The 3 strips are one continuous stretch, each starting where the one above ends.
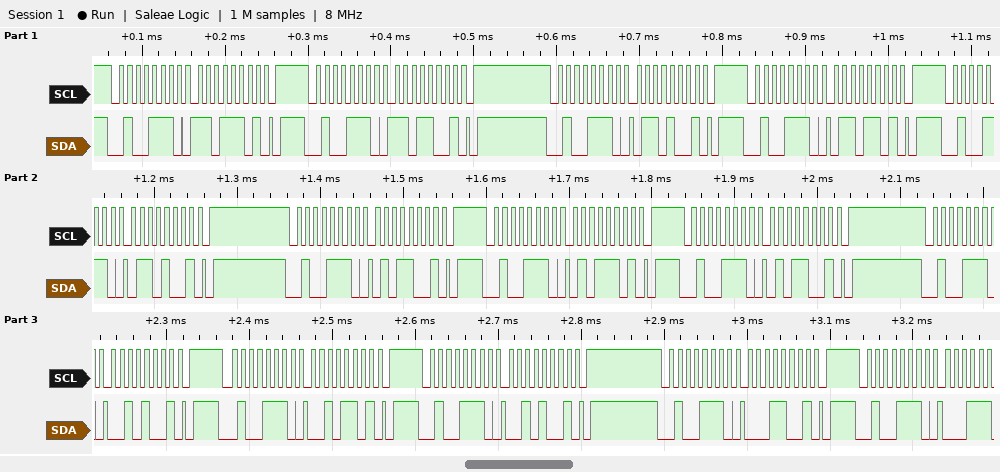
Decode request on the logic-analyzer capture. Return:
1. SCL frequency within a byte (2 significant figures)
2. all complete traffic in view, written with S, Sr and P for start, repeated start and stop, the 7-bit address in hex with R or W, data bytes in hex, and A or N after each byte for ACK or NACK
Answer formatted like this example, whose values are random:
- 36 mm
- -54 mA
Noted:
- 100 kHz
- S 27W A DD A P S 27W A D9 A P S 27W A 69 A P S 27W A 6D A P S 27W A 69 A P S 27W A 59 A P S 27W A 5D A P S 27W A 59 A P S 27W A 29 A P S 27W A 2D A P S 27W A 29 A P S 27W A 19 A P S 27W A
